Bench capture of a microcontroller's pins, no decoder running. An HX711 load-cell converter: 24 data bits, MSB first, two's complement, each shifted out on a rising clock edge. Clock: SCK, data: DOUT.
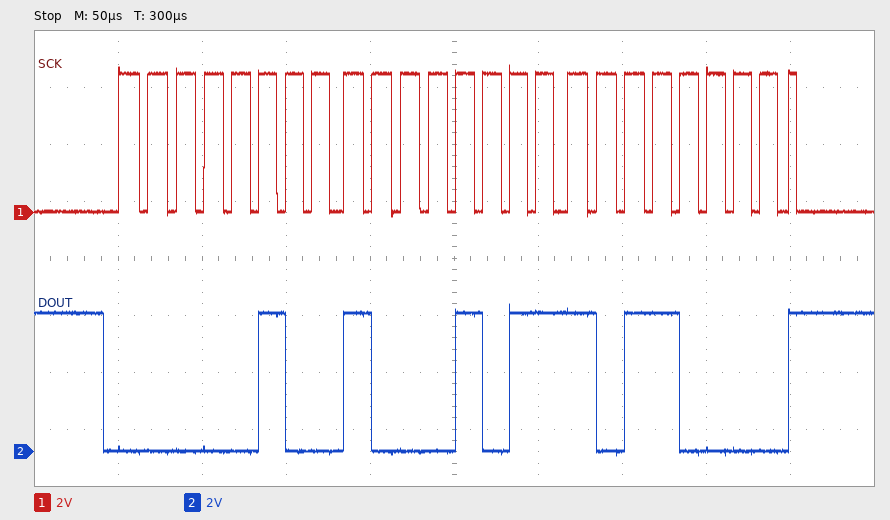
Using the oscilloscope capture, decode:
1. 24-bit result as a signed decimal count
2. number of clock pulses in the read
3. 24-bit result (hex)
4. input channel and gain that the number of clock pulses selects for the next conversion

297904
25
0x048BB0
channel A, gain 128
